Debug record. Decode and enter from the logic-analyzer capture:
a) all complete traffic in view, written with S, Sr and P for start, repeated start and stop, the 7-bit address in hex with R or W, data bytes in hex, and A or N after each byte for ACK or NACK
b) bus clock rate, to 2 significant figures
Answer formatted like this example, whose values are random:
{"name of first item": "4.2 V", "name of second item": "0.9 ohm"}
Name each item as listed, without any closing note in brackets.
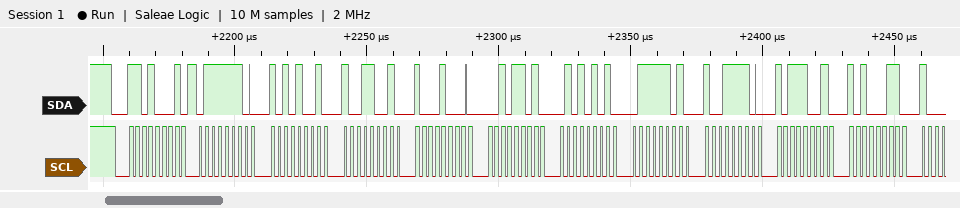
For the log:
{"all complete traffic in view, written with S, Sr and P for start, repeated start and stop, the 7-bit address in hex with R or W, data bytes in hex, and A or N after each byte for ACK or NACK": "S 68R A 7E A A9 A 99 A 88 A 2D A 55 A 7D A 9E A B9 A A3 A", "bus clock rate, to 2 significant figures": "400 kHz"}
